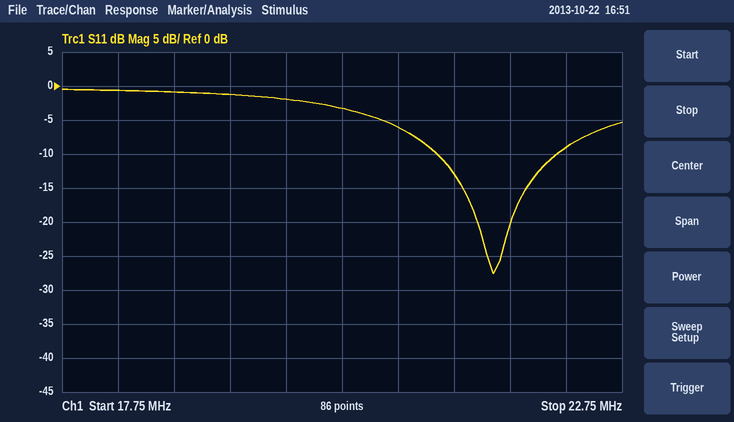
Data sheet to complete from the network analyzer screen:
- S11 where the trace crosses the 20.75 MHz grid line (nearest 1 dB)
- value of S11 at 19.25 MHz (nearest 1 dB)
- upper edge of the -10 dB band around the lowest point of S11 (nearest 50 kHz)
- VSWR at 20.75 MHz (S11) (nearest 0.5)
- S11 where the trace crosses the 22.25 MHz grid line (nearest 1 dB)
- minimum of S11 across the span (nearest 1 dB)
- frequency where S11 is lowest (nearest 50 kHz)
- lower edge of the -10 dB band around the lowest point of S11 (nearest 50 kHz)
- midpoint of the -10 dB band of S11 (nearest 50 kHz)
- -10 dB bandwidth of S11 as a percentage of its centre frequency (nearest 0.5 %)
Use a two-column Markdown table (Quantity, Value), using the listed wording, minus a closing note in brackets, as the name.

| Quantity | Value |
|---|---|
| S11 where the trace crosses the 20.75 MHz grid line | -6 dB |
| value of S11 at 19.25 MHz | -1 dB |
| upper edge of the -10 dB band around the lowest point of S11 | 22.15 MHz |
| VSWR at 20.75 MHz (S11) | 3.0 |
| S11 where the trace crosses the 22.25 MHz grid line | -9 dB |
| minimum of S11 across the span | -28 dB |
| frequency where S11 is lowest | 21.60 MHz |
| lower edge of the -10 dB band around the lowest point of S11 | 21.10 MHz |
| midpoint of the -10 dB band of S11 | 21.65 MHz |
| -10 dB bandwidth of S11 as a percentage of its centre frequency | 5.0 % |
